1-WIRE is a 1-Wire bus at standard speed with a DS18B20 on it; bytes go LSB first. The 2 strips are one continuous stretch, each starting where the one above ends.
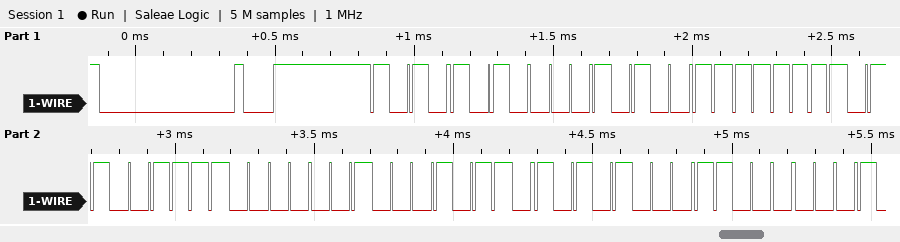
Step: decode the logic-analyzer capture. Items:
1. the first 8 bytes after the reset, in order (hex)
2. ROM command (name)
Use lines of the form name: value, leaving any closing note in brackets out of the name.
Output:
the first 8 bytes after the reset, in order: 55 28 FF E6 81 68 15 03
ROM command: Match ROM
